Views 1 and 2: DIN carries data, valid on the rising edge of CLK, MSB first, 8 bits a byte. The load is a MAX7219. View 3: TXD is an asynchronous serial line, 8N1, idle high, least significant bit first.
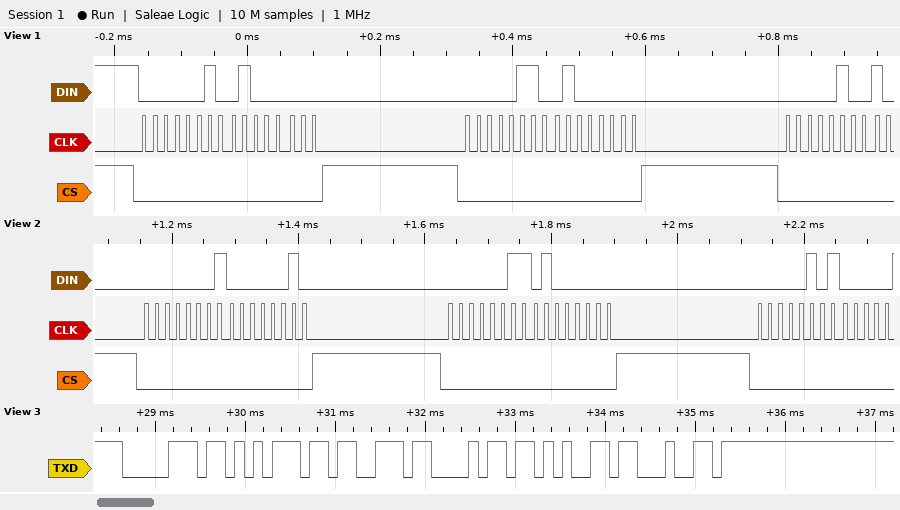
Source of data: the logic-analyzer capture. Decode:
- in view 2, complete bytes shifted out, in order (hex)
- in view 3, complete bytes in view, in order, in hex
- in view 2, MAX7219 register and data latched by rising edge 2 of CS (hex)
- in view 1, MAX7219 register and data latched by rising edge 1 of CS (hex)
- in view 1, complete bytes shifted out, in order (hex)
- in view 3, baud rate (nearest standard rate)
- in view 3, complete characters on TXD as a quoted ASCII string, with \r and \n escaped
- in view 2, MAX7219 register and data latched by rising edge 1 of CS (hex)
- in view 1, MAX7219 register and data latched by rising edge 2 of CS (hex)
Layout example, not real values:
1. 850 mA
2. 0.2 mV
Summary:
1. 01 02 03 40 05
2. 70 75 73 68 65 64
3. register 0x3, data 0x40
4. register 0x2, data 0x40
5. 0x02 0x40 0x06 0x40 0x04
6. 9600 baud
7. "pushed"
8. register 0x1, data 0x02
9. register 0x6, data 0x40
